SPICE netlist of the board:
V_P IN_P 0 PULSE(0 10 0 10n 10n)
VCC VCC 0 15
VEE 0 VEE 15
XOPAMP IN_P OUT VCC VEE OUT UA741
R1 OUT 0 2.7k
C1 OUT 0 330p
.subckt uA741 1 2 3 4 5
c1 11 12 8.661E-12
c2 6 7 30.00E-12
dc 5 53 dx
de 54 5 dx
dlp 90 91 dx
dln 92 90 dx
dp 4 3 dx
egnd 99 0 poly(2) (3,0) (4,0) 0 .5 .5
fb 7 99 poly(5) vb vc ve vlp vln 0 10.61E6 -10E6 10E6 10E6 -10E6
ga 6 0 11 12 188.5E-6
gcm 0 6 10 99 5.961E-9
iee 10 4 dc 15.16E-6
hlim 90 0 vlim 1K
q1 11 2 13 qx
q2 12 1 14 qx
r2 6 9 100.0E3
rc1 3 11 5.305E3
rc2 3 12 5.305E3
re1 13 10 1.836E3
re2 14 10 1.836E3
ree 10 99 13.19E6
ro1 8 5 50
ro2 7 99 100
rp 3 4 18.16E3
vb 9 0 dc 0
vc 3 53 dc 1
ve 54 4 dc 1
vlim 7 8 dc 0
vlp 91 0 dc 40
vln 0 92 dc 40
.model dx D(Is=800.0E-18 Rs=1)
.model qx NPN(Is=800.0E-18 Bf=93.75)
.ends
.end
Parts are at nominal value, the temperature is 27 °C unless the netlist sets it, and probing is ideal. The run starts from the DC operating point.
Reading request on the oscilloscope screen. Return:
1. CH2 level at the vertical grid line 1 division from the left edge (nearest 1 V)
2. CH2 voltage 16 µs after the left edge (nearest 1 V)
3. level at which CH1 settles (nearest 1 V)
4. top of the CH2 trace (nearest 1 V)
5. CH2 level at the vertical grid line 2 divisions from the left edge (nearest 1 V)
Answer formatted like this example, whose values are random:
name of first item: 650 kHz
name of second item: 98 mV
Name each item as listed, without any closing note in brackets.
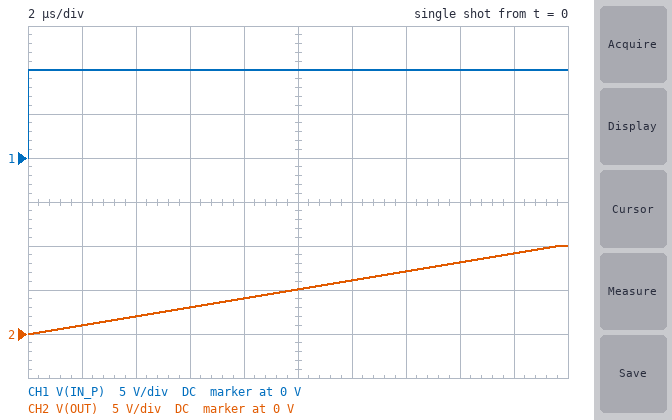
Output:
CH2 level at the vertical grid line 1 division from the left edge: 1 V
CH2 voltage 16 µs after the left edge: 8 V
level at which CH1 settles: 10 V
top of the CH2 trace: 10 V
CH2 level at the vertical grid line 2 divisions from the left edge: 2 V
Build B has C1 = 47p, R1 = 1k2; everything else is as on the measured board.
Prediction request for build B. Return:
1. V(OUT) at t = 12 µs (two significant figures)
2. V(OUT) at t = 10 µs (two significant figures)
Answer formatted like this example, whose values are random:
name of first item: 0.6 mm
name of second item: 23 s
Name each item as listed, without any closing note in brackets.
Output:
V(OUT) at t = 12 µs: 6.0 V
V(OUT) at t = 10 µs: 5.0 V
